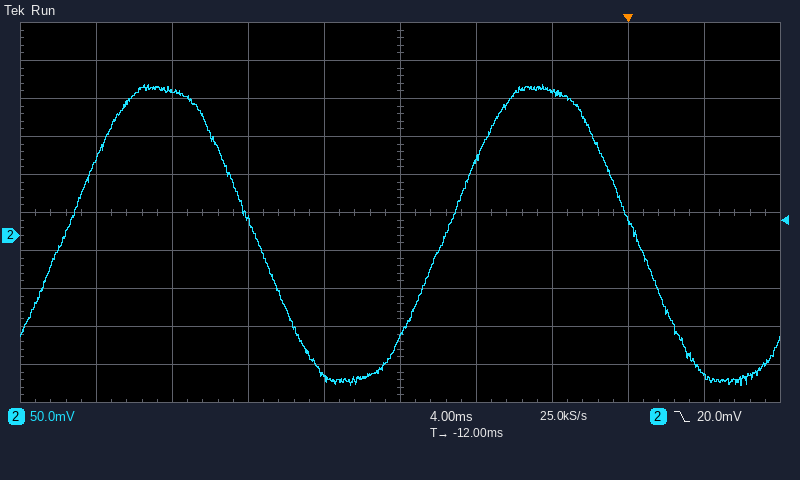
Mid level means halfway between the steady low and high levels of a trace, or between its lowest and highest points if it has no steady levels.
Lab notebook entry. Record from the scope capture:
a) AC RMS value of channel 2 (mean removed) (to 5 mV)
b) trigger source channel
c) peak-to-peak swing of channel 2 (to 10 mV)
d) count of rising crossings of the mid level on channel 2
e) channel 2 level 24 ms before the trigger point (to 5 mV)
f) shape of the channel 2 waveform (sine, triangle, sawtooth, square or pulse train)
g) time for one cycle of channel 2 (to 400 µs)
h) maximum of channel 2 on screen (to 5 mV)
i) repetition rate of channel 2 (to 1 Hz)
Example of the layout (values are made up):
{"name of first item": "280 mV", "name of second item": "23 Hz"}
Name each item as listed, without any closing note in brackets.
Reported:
{"AC RMS value of channel 2 (mean removed)": "140 mV", "trigger source channel": "channel 2", "peak-to-peak swing of channel 2": "400 mV", "count of rising crossings of the mid level on channel 2": "2", "channel 2 level 24 ms before the trigger point": "190 mV", "shape of the channel 2 waveform": "sine", "time for one cycle of channel 2": "20.0 ms", "maximum of channel 2 on screen": "200 mV", "repetition rate of channel 2": "50 Hz"}
